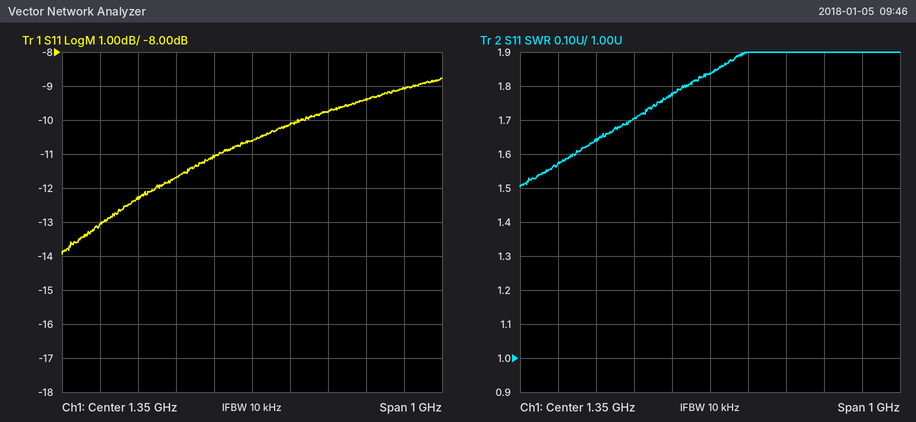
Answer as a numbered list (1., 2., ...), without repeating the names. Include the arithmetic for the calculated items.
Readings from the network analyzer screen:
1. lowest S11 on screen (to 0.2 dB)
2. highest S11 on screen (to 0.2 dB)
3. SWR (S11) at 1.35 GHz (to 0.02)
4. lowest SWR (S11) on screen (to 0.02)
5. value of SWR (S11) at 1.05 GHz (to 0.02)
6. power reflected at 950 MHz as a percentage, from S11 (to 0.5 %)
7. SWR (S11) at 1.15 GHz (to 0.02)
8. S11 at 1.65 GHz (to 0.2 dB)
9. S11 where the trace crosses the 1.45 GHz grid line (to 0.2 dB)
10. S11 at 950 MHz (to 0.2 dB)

1. -14.0 dB
2. -8.8 dB
3. 1.84
4. 1.50
5. 1.64
6. 10^(-13/10) ≈ 5.0 %
7. 1.70
8. -9.4 dB
9. -10.2 dB
10. -13.0 dB
